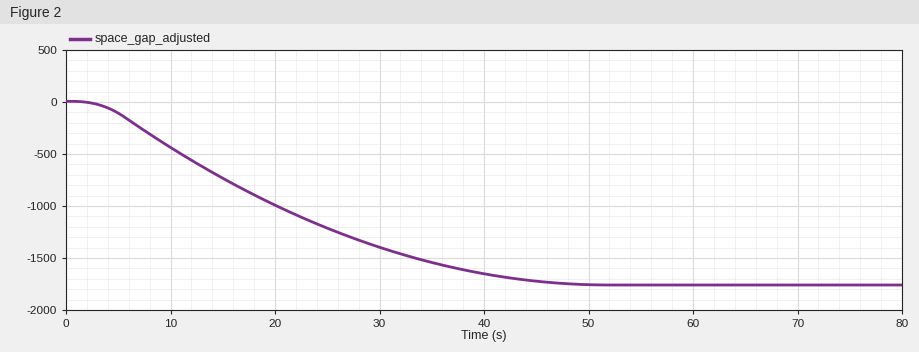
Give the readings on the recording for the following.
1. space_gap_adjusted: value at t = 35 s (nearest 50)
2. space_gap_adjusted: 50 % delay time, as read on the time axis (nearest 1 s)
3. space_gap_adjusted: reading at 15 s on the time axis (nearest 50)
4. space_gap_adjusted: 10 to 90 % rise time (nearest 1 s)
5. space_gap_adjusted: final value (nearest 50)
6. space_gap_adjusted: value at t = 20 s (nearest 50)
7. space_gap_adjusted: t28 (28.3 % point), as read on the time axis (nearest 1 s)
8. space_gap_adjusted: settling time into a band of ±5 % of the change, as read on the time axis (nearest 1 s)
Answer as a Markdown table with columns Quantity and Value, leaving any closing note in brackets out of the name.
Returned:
| Quantity | Value |
|---|---|
| space_gap_adjusted: value at t = 35 s | -1550 |
| space_gap_adjusted: 50 % delay time, as read on the time axis | 18 s |
| space_gap_adjusted: reading at 15 s on the time axis | -750 |
| space_gap_adjusted: 10 to 90 % rise time | 31 s |
| space_gap_adjusted: final value | -1750 |
| space_gap_adjusted: value at t = 20 s | -1000 |
| space_gap_adjusted: t28 (28.3 % point), as read on the time axis | 11 s |
| space_gap_adjusted: settling time into a band of ±5 % of the change, as read on the time axis | 41 s |
